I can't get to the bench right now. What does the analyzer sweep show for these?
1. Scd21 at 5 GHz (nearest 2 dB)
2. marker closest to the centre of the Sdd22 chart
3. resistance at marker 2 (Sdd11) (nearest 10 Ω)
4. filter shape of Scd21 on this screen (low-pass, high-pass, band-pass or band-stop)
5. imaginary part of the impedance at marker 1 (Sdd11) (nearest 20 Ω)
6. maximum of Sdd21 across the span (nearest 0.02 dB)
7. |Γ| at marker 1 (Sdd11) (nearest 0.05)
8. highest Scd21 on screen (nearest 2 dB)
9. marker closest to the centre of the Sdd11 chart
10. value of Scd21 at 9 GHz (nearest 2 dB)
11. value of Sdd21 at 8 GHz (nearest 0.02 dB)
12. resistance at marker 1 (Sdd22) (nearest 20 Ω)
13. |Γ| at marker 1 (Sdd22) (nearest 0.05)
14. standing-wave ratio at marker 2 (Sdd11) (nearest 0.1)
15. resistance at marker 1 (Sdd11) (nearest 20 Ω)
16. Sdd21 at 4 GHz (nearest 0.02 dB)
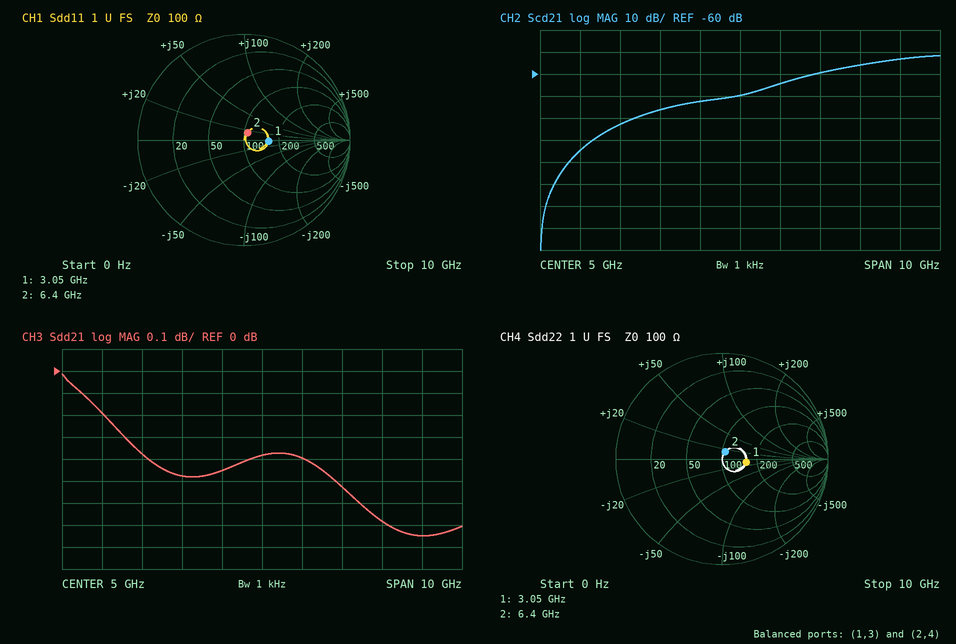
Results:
-70 dB
marker 2
110 Ω
high-pass
0 Ω
-0.02 dB
0.25
-52 dB
marker 2
-54 dB
-0.68 dB
160 Ω
0.25
1.2
160 Ω
-0.46 dB
